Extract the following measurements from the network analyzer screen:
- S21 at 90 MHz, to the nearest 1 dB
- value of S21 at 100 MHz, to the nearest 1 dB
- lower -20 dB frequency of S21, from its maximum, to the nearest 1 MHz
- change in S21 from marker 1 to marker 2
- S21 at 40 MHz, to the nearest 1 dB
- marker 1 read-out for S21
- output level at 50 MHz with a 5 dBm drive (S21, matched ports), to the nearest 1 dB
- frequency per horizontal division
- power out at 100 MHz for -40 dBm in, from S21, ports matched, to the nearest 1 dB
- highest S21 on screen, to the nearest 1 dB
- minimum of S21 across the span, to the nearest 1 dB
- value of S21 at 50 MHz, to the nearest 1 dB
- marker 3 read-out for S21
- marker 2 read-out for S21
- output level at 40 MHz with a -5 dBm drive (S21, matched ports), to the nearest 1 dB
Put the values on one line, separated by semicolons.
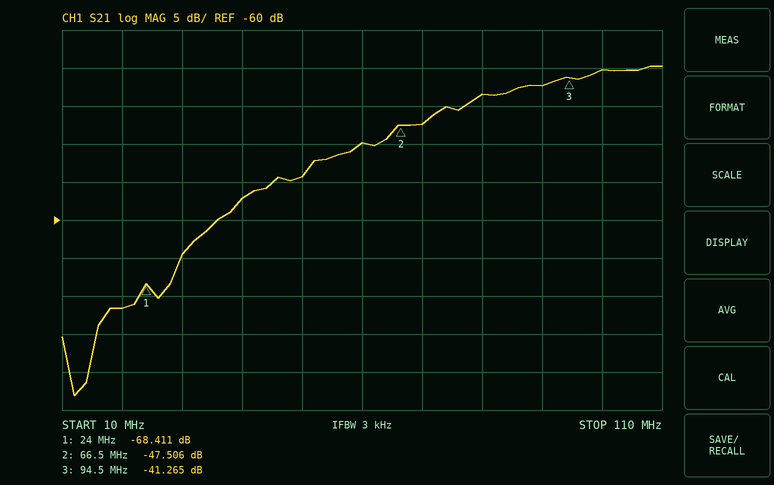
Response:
-42 dB; -40 dB; 36 MHz; 20.905 dB; -57 dB; -68.411 dB; -49 dBm; 10 MHz; -80 dBm; -40 dB; -83 dB; -54 dB; -41.265 dB; -47.506 dB; -62 dBm
